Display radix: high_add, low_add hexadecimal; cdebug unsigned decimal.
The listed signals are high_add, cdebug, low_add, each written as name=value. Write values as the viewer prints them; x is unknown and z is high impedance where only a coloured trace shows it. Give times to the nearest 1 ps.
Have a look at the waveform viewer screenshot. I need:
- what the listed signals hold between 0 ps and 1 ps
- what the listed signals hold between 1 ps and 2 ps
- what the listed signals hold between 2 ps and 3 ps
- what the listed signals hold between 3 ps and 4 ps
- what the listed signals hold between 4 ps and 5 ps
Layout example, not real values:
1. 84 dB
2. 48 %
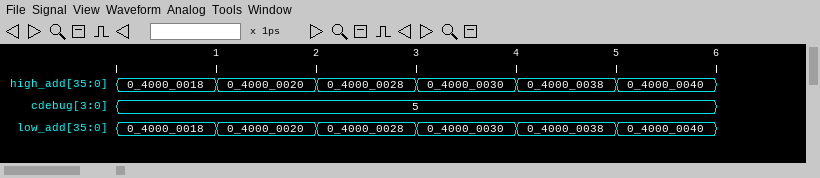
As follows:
1. high_add=0_4000_0018, cdebug=5, low_add=0_4000_0018
2. high_add=0_4000_0020, cdebug=5, low_add=0_4000_0020
3. high_add=0_4000_0028, cdebug=5, low_add=0_4000_0028
4. high_add=0_4000_0030, cdebug=5, low_add=0_4000_0030
5. high_add=0_4000_0038, cdebug=5, low_add=0_4000_0038
